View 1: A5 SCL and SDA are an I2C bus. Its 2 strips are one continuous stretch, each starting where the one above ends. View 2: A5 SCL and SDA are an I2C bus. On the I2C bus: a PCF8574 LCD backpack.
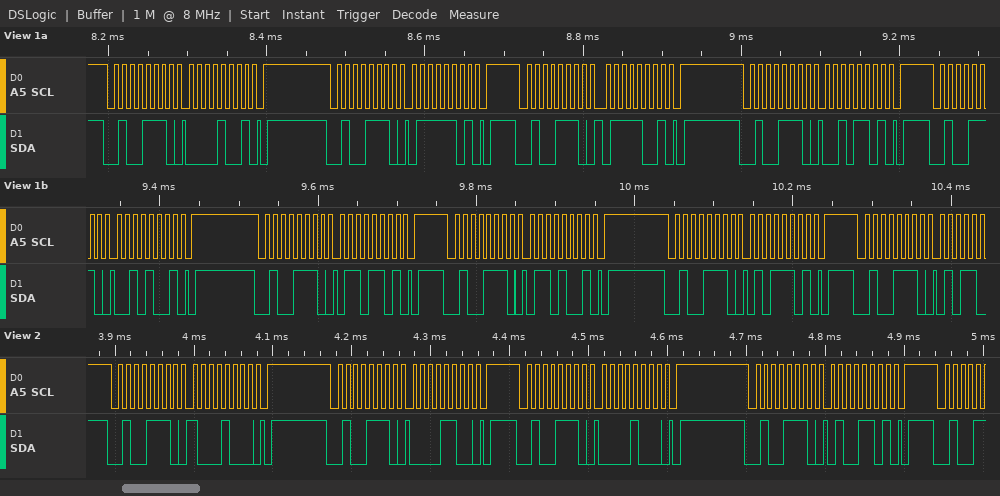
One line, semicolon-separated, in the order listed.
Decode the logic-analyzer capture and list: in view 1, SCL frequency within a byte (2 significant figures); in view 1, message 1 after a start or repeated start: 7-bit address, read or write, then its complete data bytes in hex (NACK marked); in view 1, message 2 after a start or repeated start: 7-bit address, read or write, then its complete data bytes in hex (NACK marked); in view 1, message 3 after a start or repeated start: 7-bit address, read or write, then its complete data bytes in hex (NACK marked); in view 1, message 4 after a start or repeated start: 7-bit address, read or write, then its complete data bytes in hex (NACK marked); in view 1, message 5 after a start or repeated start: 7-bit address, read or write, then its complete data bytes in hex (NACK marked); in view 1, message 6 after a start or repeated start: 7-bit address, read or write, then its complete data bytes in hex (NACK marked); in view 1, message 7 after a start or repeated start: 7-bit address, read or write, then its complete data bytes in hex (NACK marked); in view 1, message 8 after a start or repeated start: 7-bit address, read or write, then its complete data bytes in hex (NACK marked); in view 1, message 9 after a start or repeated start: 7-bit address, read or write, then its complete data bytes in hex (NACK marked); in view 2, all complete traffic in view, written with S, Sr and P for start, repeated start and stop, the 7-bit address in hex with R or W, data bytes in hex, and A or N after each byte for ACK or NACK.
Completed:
100 kHz; 0x27 write: 09; 0x27 write: 7D; 0x27 write: 79; 0x27 write: 2D; 0x27 write: 29; 0x27 write: 6D; 0x27 write: 69; 0x27 write: 5D; 0x27 write; S 27W A 88 A P S 27W A 0C A P S 27W A 08 A P S 27W A 4D A P
